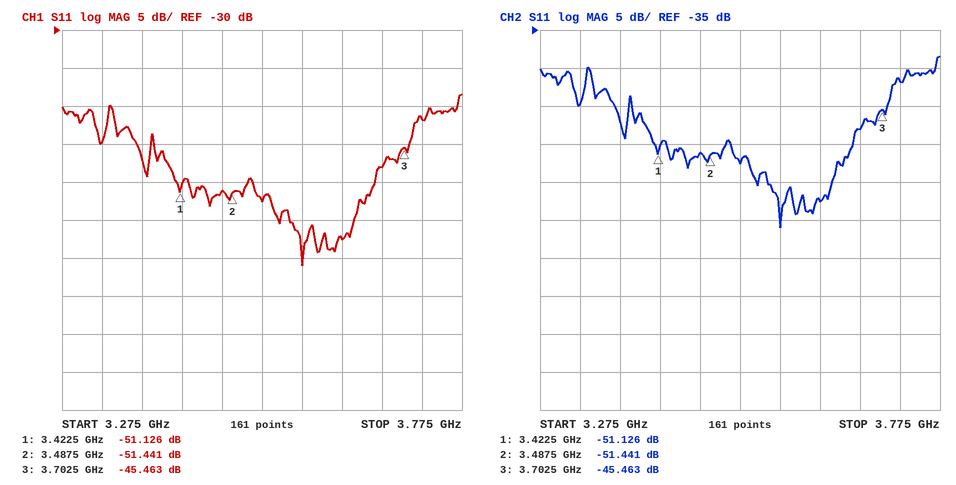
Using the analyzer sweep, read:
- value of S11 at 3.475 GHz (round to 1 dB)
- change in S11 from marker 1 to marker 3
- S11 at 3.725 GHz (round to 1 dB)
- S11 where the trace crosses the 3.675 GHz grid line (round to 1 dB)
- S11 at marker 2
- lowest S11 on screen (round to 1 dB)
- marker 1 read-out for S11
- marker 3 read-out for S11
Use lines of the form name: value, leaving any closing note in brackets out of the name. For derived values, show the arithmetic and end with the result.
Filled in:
value of S11 at 3.475 GHz: -51 dB
change in S11 from marker 1 to marker 3: -45.463 − (-51.126) = 5.663 dB
S11 at 3.725 GHz: -42 dB
S11 where the trace crosses the 3.675 GHz grid line: -48 dB
S11 at marker 2: -51.441 dB
lowest S11 on screen: -61 dB
marker 1 read-out for S11: -51.126 dB
marker 3 read-out for S11: -45.463 dB
